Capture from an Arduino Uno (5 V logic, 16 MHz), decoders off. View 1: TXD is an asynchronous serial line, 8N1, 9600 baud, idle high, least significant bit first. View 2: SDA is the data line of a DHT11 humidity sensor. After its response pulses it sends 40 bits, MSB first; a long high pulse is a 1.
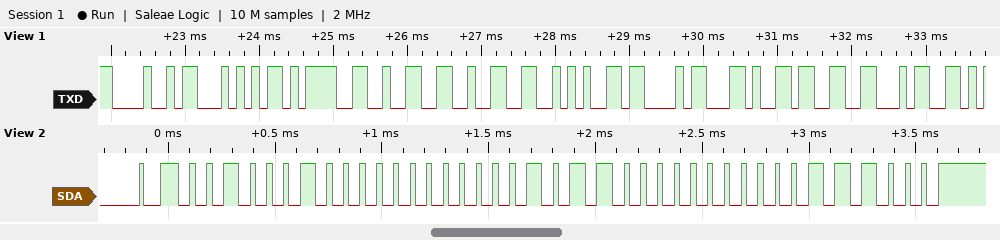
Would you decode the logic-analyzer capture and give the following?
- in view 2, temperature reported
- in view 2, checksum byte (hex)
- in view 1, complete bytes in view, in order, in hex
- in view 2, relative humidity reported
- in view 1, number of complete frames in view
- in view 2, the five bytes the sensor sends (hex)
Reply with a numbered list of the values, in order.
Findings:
1. 22.0 °C
2. 0x38
3. 0x48 0x54 0x3D 0x32 0x32 0x2A 0x43 0x2C 0x33 0x34
4. 34 %
5. 10
6. 22 00 16 00 38
